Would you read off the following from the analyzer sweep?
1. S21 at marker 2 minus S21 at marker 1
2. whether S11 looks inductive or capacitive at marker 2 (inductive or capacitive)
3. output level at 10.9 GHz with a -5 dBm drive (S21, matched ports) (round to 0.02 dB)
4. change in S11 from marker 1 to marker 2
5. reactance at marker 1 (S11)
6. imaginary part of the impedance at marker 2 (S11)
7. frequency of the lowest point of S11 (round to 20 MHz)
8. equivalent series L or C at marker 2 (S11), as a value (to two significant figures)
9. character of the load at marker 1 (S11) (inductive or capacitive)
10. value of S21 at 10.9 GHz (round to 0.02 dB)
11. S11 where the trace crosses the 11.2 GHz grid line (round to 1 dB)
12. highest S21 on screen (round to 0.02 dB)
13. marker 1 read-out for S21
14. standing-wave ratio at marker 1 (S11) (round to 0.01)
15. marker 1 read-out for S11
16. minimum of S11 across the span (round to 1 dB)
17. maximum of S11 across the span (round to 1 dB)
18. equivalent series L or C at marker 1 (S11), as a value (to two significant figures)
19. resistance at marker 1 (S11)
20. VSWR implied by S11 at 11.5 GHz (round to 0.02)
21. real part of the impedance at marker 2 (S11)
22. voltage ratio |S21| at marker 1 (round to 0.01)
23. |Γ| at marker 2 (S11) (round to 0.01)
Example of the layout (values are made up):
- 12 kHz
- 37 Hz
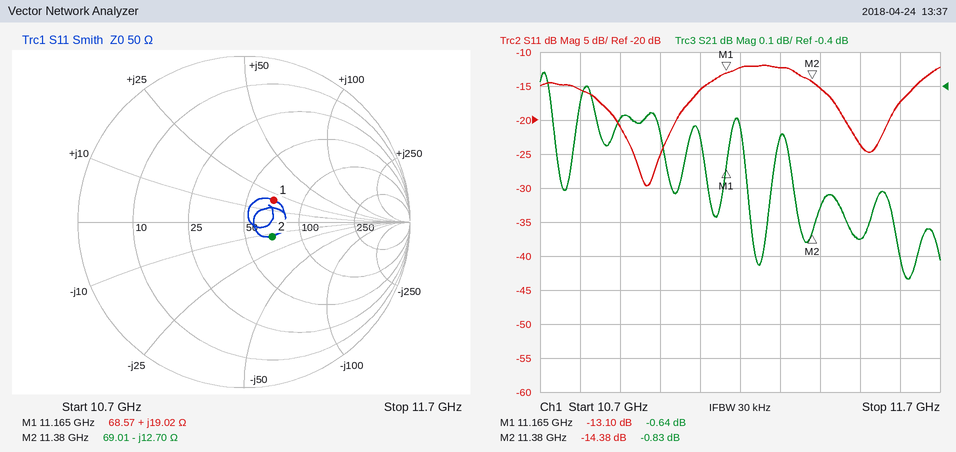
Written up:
- -0.19 dB
- capacitive
- -5.50 dBm
- -1.28 dB
- +19.02 Ω
- -12.70 Ω
- 10.96 GHz
- 1.1 pF
- inductive
- -0.50 dB
- -12 dB
- -0.36 dB
- -0.64 dB
- 1.57
- -13.10 dB
- -30 dB
- -12 dB
- 270 pH
- 68.57 Ω
- 1.14
- 69.01 Ω
- 0.93
- 0.19
